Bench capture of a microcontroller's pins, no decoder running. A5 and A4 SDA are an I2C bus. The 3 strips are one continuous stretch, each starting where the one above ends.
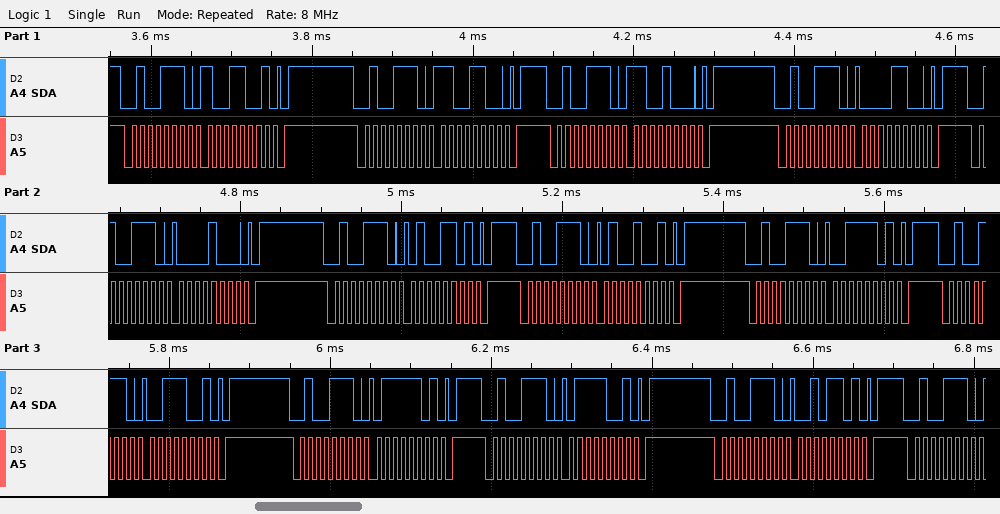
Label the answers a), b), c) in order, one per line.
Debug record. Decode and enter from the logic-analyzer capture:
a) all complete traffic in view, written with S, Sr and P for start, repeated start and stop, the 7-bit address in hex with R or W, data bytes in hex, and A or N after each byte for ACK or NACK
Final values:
a) S 27W A 99 A P S 27W A CC A P S 27W A C8 A P S 27W A 0C A P S 27W A 08 A P S 27W A 4D A P S 27W A 49 A P S 27W A 3D A P S 27W A 39 A P S 27W A 7D A P S 27W A 79 A P S 27W A 2D A P S 27W A
